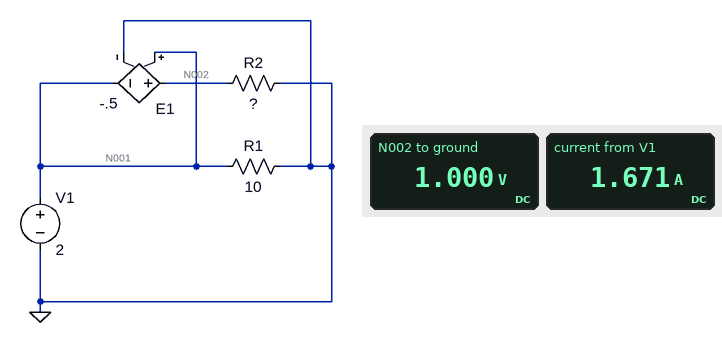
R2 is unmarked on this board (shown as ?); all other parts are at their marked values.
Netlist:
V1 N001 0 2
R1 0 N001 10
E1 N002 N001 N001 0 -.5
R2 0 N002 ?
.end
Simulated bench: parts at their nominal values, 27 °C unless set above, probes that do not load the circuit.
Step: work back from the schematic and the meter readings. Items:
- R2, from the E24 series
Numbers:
0.68 Ω
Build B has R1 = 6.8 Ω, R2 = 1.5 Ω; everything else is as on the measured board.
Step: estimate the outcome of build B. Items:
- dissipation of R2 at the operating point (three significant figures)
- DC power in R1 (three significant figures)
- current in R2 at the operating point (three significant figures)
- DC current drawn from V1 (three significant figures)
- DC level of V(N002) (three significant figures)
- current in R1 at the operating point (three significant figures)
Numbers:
667 mW
588 mW
667 mA
961 mA
1.00 V
294 mA
